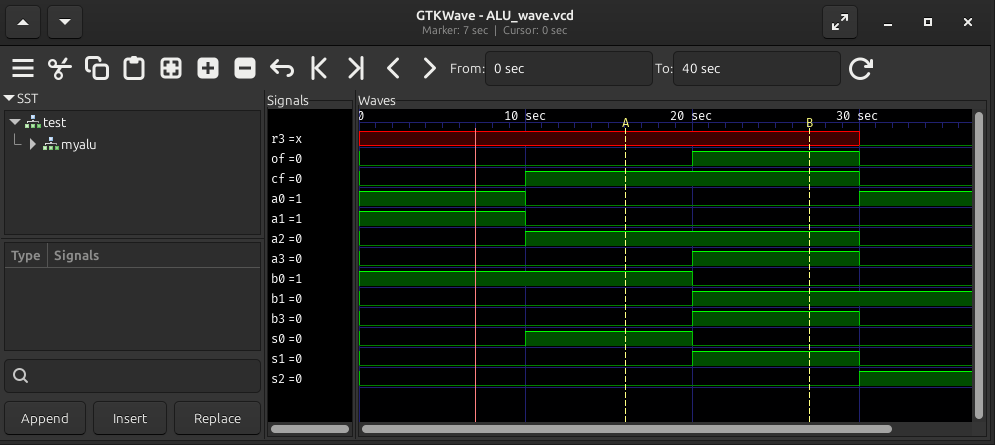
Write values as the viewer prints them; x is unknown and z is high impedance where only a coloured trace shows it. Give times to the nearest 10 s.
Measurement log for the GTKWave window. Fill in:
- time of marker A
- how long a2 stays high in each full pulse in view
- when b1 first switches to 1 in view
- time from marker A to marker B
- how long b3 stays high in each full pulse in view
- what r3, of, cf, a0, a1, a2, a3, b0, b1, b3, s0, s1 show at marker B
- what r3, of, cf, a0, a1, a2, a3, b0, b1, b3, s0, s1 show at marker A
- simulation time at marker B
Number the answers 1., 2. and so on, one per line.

1. 20 s
2. 20 s
3. 20 s
4. 10 s
5. 10 s
6. r3=x, of=1, cf=1, a0=0, a1=0, a2=1, a3=1, b0=0, b1=1, b3=1, s0=0, s1=1
7. r3=x, of=0, cf=1, a0=0, a1=0, a2=1, a3=0, b0=1, b1=0, b3=0, s0=1, s1=0
8. 30 s
